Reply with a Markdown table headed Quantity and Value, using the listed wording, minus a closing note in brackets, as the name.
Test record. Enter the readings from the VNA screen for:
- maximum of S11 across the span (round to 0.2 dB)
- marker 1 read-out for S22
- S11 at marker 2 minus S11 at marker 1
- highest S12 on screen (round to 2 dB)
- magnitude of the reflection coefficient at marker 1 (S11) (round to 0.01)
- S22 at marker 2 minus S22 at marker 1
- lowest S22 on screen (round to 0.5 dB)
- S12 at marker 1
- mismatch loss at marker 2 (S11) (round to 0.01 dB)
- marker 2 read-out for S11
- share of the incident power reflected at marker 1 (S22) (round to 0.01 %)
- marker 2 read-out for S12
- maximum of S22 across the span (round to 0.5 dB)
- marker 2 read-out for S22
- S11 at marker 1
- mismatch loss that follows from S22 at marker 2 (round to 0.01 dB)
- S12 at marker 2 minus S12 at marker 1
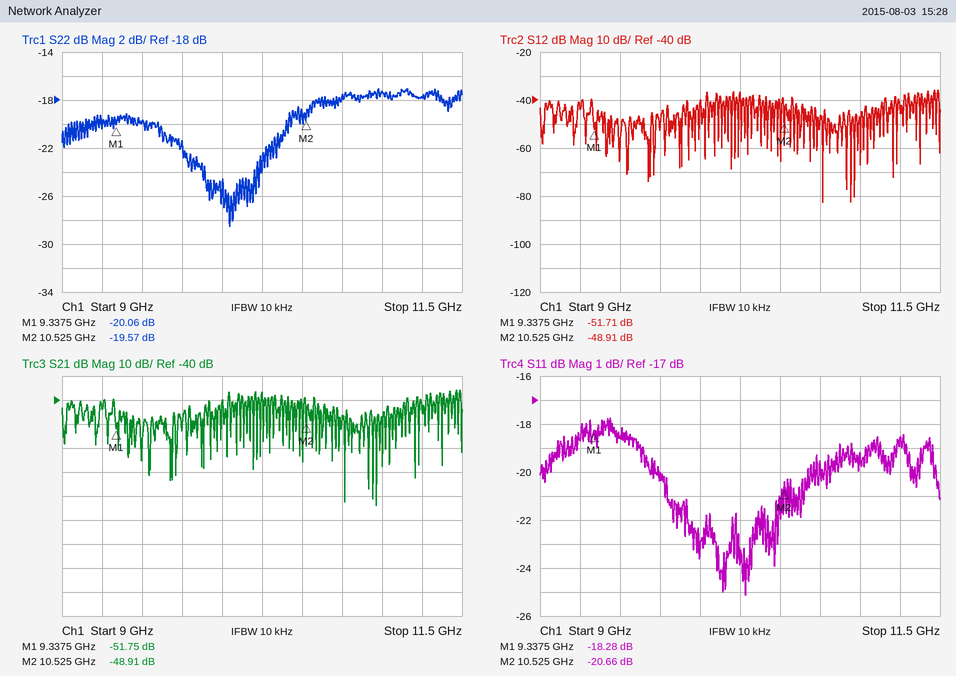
| Quantity | Value |
|---|---|
| maximum of S11 across the span | -17.8 dB |
| marker 1 read-out for S22 | -20.06 dB |
| S11 at marker 2 minus S11 at marker 1 | -2.38 dB |
| highest S12 on screen | -36 dB |
| magnitude of the reflection coefficient at marker 1 (S11) | 0.12 |
| S22 at marker 2 minus S22 at marker 1 | 0.49 dB |
| lowest S22 on screen | -28.5 dB |
| S12 at marker 1 | -51.71 dB |
| mismatch loss at marker 2 (S11) | 0.04 dB |
| marker 2 read-out for S11 | -20.66 dB |
| share of the incident power reflected at marker 1 (S22) | 0.99 % |
| marker 2 read-out for S12 | -48.91 dB |
| maximum of S22 across the span | -17.0 dB |
| marker 2 read-out for S22 | -19.57 dB |
| S11 at marker 1 | -18.28 dB |
| mismatch loss that follows from S22 at marker 2 | 0.05 dB |
| S12 at marker 2 minus S12 at marker 1 | 2.80 dB |
